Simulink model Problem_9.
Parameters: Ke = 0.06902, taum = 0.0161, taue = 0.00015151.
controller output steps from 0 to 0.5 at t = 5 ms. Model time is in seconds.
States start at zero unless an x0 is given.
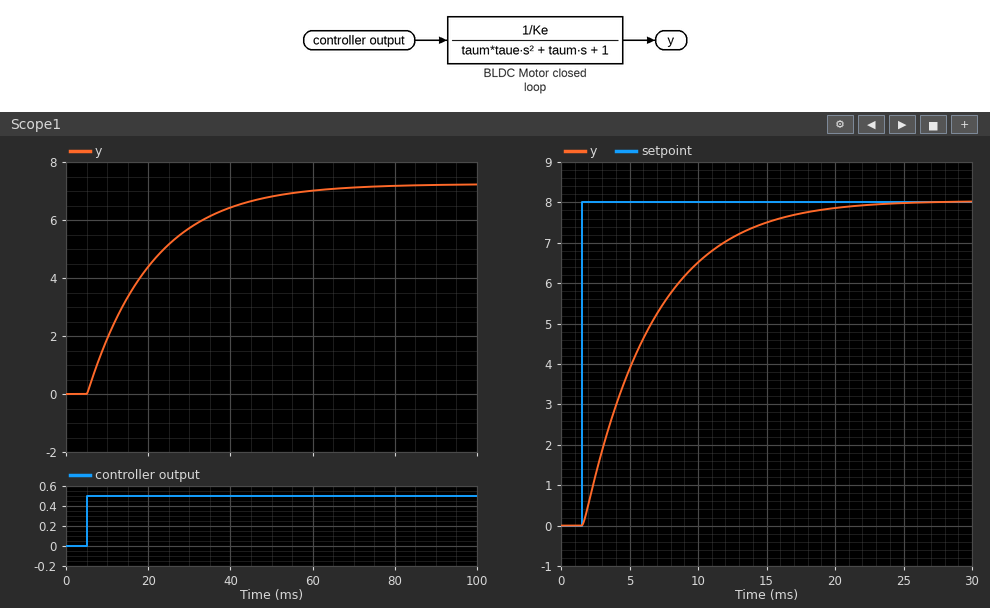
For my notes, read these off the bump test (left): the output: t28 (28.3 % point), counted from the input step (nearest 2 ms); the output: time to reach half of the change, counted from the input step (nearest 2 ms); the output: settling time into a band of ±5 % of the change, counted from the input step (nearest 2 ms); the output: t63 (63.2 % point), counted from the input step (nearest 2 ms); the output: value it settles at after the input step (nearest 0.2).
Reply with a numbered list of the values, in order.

1. 6 ms
2. 12 ms
3. 48 ms
4. 16 ms
5. 7.2
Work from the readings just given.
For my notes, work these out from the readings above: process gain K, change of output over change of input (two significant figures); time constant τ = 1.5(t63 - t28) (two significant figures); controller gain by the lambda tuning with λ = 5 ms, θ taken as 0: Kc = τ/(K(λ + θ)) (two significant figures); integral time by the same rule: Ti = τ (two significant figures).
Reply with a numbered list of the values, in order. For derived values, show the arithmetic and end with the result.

1. (7.2 - 0) / 0.5 = 14
2. 1.5 × (16 - 6) = 15 ms
3. 15 / (14 × (5 + 0)) = 0.21
4. 15 ms
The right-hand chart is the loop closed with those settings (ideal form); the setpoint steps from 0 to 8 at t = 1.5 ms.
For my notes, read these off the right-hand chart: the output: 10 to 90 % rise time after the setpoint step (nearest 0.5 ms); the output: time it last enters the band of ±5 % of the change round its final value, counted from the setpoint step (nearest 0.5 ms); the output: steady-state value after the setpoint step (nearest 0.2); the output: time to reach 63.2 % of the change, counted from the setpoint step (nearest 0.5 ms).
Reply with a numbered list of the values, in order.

1. 10.5 ms
2. 14.5 ms
3. 8.0
4. 5.0 ms
